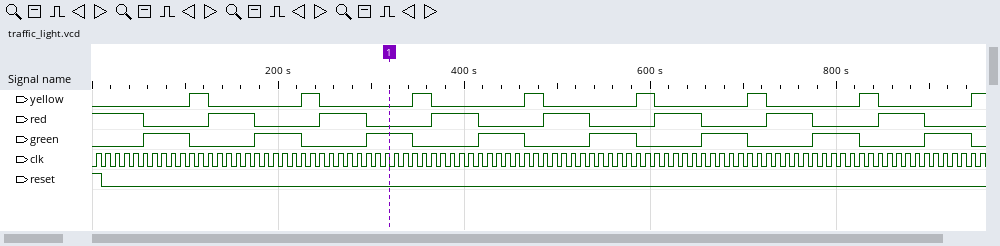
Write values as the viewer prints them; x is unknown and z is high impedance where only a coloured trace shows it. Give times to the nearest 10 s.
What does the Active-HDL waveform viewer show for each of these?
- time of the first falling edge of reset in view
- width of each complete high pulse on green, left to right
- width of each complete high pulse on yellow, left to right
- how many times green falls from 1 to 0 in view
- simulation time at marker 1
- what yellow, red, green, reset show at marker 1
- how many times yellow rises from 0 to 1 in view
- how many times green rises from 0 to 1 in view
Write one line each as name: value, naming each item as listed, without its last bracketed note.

time of the first falling edge of reset in view: 10 s
width of each complete high pulse on green, left to right: 50 s, 50 s, 50 s, 50 s, 50 s, 50 s, 50 s, 50 s
width of each complete high pulse on yellow, left to right: 20 s, 20 s, 20 s, 20 s, 20 s, 20 s, 20 s
how many times green falls from 1 to 0 in view: 8
simulation time at marker 1: 320 s
what yellow, red, green, reset show at marker 1: yellow=0, red=0, green=1, reset=0
how many times yellow rises from 0 to 1 in view: 8
how many times green rises from 0 to 1 in view: 8
